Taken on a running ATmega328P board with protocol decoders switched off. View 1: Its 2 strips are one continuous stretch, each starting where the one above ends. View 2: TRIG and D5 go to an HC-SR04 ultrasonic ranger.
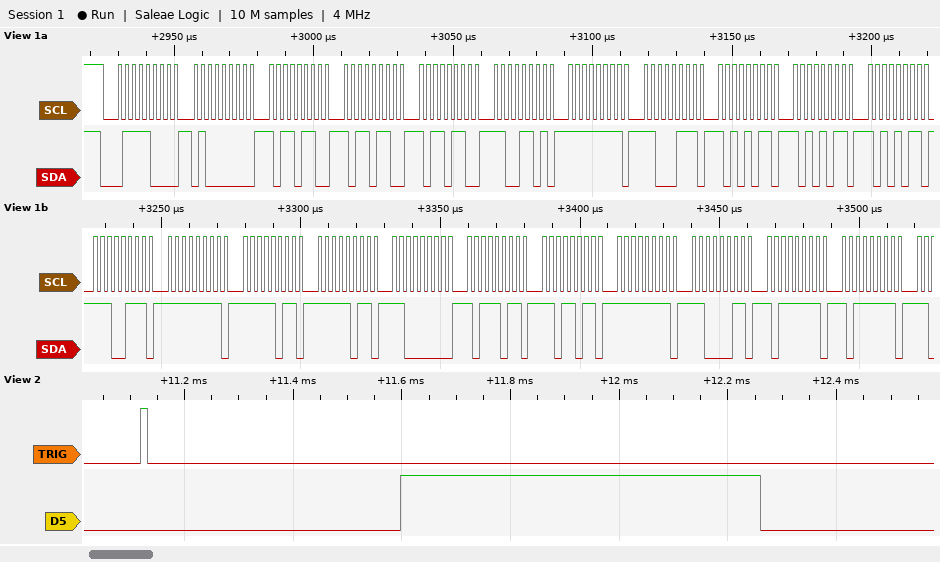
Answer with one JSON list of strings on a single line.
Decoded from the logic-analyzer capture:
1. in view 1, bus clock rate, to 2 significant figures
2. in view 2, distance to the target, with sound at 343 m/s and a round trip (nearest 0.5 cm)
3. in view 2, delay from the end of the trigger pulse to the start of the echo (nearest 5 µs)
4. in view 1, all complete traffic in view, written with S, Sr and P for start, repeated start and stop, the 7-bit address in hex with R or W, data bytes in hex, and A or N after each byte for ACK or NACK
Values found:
["400 kHz", "11.5 cm", "465 µs", "S 3CW A 40 A B6 A B6 A B6 A CD A FF A C7 A AB A AB A AB A E7 A FF A FB A FB A C0 A BB A DB A FF A C3 A BF A BF A"]
